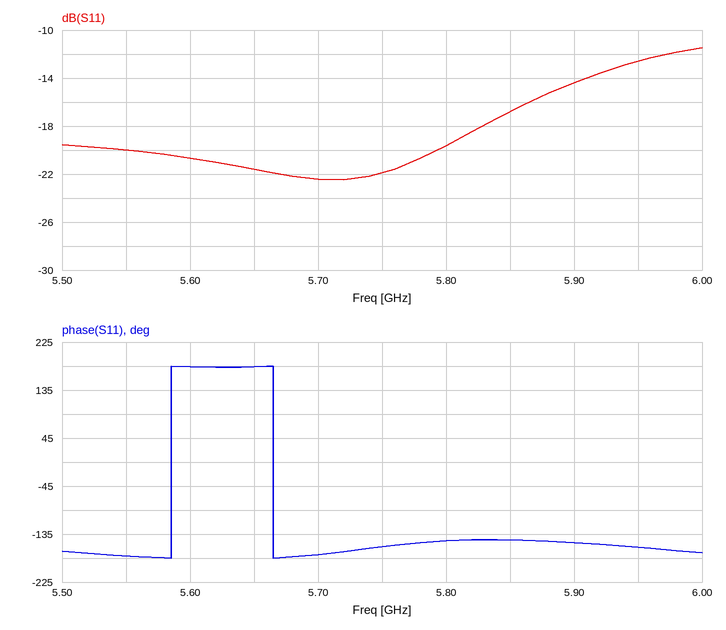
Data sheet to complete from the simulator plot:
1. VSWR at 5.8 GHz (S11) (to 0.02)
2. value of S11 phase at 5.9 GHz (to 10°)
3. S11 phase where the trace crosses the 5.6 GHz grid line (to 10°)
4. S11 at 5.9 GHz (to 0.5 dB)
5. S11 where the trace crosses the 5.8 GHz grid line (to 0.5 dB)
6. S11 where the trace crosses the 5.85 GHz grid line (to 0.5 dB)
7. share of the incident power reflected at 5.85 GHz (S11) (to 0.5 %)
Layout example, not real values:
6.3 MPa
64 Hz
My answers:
1.24
-150°
180°
-14.5 dB
-19.5 dB
-17.0 dB
2.0 %
